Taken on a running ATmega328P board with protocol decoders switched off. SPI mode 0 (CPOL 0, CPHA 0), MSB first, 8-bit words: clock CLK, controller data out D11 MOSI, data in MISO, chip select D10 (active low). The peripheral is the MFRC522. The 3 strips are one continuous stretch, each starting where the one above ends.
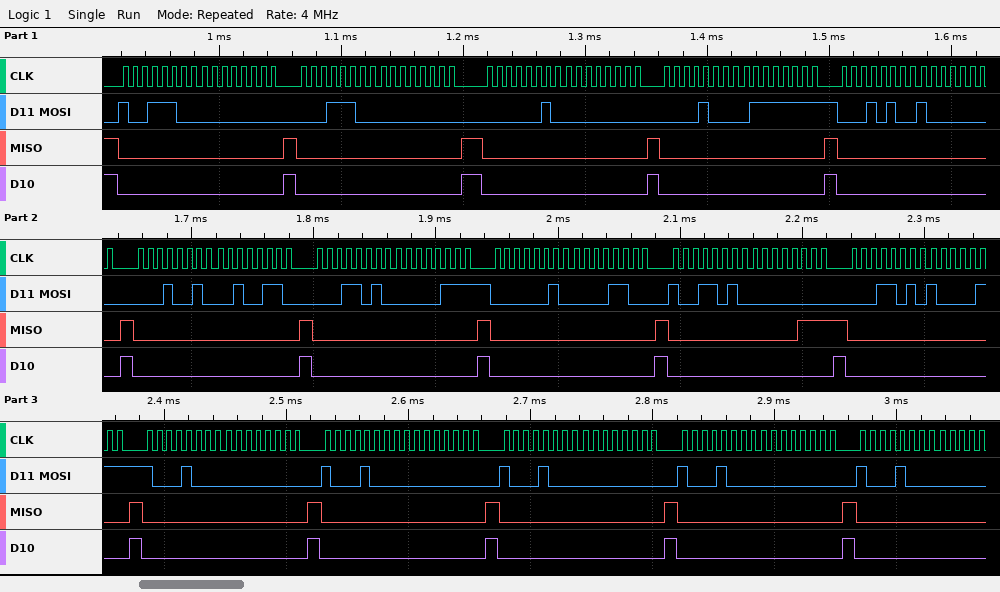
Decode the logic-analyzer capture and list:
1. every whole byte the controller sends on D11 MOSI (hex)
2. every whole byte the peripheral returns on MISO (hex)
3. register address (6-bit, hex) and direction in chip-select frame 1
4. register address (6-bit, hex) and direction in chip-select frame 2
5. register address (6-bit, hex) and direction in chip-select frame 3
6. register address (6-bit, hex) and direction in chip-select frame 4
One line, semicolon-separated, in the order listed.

9C 00 1C 00 02 00 08 7F 14 80 12 26 1A 07 02 0C 9A 00 1A 87 88 00 88 00 88 00 88 00 88; 00 00 00 00 00 00 00 00 00 00 00 00 00 00 00 00 00 07 00 00 00 00 00 00 00 00 00 00 00; 0x0E read; 0x0E write; 0x01 write; 0x04 write
